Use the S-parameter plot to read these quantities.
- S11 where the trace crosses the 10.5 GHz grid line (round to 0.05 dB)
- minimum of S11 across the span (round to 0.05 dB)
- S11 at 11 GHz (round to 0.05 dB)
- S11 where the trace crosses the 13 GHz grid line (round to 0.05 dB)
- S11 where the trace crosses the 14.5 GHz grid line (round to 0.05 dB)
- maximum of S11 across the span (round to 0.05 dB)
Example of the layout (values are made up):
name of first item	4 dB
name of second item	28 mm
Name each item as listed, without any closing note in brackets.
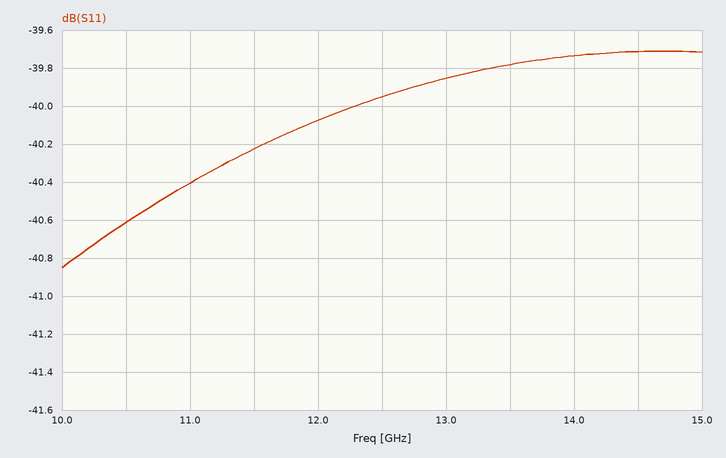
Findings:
S11 where the trace crosses the 10.5 GHz grid line	-40.60 dB
minimum of S11 across the span	-40.85 dB
S11 at 11 GHz	-40.40 dB
S11 where the trace crosses the 13 GHz grid line	-39.85 dB
S11 where the trace crosses the 14.5 GHz grid line	-39.70 dB
maximum of S11 across the span	-39.70 dB
